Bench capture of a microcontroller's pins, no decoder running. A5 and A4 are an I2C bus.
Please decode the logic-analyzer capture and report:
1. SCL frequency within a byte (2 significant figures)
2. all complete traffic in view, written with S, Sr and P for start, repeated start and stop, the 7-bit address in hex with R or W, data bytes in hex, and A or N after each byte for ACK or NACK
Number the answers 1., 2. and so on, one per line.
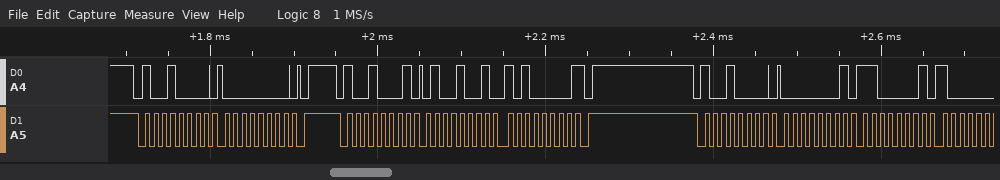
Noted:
1. 100 kHz
2. S 48W A 00 A P S 48R A 49 A A0 N P S 48W A 01 A C1 A
